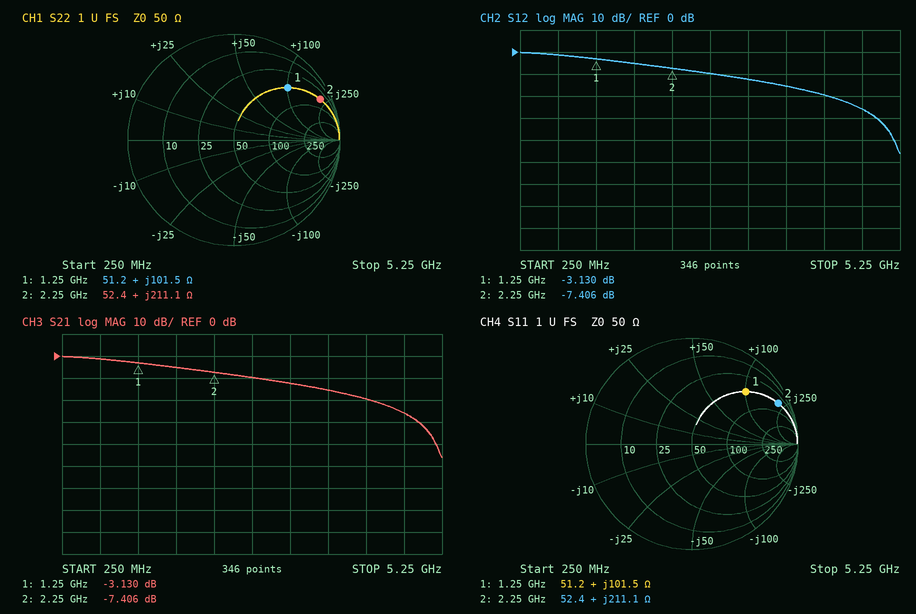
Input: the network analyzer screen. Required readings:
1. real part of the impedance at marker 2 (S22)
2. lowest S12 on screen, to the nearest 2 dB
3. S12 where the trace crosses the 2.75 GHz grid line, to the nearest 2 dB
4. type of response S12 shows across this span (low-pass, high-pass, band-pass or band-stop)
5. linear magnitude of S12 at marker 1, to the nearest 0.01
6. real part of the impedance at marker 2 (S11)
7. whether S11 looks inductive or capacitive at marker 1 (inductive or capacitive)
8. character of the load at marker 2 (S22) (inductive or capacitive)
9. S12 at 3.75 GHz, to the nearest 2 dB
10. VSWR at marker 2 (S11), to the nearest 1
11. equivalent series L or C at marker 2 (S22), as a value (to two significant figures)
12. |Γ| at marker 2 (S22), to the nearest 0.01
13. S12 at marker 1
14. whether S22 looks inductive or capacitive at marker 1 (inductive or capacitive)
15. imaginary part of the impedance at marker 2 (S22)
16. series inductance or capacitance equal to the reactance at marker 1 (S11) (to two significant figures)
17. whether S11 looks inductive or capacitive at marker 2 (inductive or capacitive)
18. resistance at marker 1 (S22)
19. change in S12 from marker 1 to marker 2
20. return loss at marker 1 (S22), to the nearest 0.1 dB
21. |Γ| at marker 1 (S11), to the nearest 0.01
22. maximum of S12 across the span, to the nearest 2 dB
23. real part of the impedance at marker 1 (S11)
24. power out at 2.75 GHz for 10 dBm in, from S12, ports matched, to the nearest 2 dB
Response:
52.4 Ω
-46 dB
-10 dB
low-pass
0.70
52.4 Ω
inductive
inductive
-16 dB
19
15 nH
0.90
-3.130 dB
inductive
+211.1 Ω
13 nH
inductive
51.2 Ω
-4.276 dB
3.0 dB
0.71
0 dB
51.2 Ω
0 dBm
